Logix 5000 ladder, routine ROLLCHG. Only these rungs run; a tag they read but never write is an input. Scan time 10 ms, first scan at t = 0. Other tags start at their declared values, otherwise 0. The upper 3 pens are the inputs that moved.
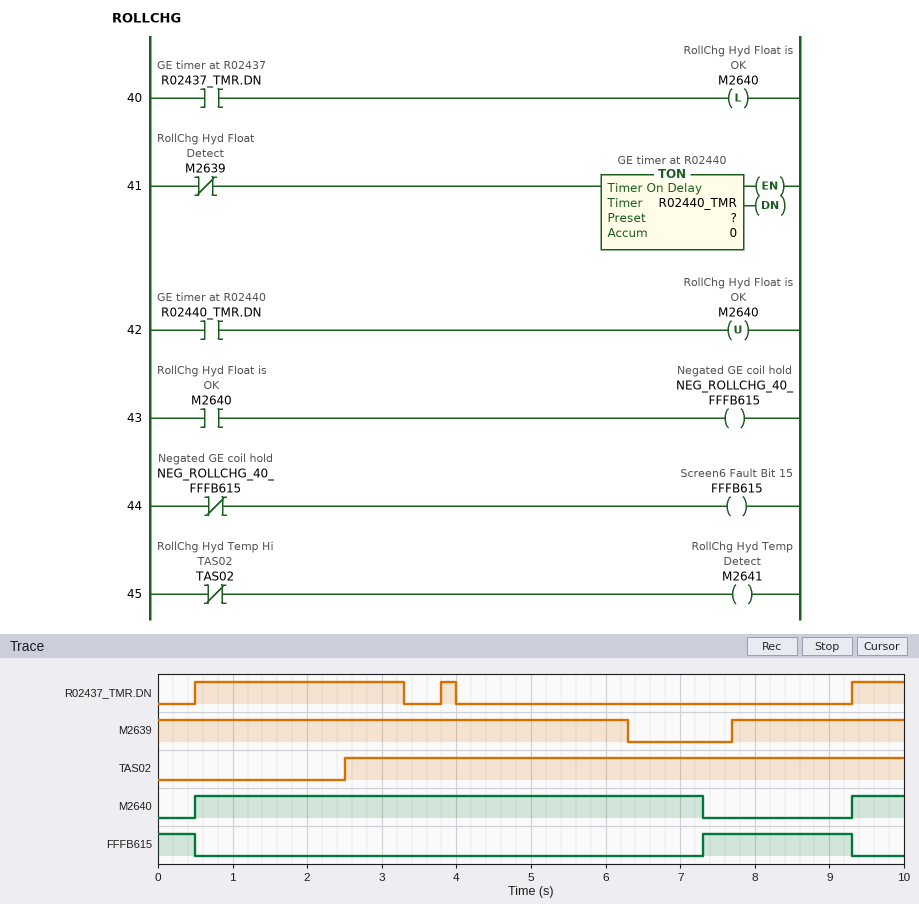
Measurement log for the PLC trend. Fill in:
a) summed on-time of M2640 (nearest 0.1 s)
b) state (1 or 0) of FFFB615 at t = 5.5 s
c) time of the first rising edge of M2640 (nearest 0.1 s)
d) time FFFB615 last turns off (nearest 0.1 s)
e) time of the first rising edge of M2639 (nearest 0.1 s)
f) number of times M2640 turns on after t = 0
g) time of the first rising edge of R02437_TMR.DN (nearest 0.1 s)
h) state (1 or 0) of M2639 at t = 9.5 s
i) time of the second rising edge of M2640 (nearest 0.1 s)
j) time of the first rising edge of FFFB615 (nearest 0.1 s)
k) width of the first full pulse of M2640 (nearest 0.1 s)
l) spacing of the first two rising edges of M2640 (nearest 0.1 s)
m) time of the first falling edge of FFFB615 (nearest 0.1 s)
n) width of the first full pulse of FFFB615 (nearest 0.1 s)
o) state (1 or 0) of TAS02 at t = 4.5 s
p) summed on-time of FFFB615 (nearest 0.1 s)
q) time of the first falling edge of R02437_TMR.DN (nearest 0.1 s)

7.5 s
0
0.5 s
9.3 s
7.7 s
2
0.5 s
1
9.3 s
7.3 s
6.8 s
8.8 s
0.5 s
2.0 s
1
2.5 s
3.3 s
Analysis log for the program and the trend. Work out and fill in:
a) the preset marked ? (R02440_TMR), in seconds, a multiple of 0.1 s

1.0 s
